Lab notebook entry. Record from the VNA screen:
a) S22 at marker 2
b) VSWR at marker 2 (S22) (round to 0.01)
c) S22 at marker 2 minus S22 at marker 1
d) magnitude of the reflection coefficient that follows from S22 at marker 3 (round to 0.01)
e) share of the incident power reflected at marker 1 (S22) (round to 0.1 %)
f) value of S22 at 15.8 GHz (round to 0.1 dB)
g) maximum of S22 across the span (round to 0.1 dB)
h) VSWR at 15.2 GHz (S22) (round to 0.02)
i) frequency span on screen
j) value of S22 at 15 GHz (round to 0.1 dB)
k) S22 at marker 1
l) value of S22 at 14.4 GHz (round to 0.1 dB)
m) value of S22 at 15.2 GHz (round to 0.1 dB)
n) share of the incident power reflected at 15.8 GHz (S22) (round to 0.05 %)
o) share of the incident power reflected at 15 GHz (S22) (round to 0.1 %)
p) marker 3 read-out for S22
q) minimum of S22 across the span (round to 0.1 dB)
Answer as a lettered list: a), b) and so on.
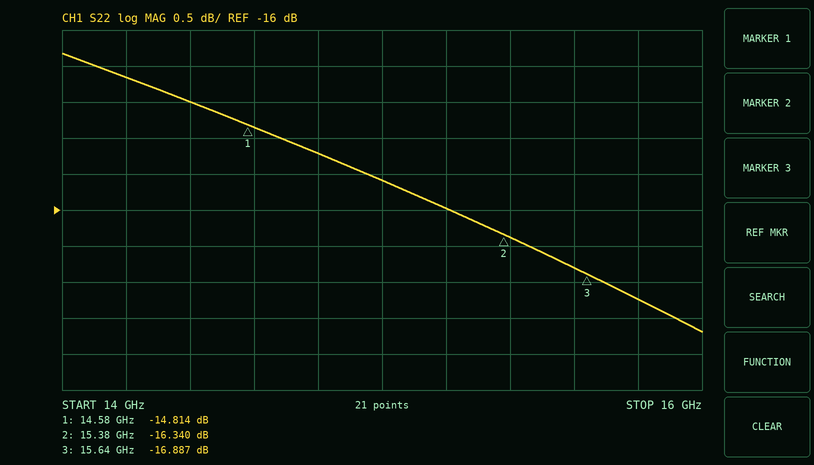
a) -16.340 dB
b) 1.36
c) -1.526 dB
d) 0.14
e) 3.3 %
f) -17.2 dB
g) -13.8 dB
h) 1.38
i) 2 GHz
j) -15.6 dB
k) -14.814 dB
l) -14.5 dB
m) -16.0 dB
n) 1.90 %
o) 2.8 %
p) -16.887 dB
q) -17.7 dB
